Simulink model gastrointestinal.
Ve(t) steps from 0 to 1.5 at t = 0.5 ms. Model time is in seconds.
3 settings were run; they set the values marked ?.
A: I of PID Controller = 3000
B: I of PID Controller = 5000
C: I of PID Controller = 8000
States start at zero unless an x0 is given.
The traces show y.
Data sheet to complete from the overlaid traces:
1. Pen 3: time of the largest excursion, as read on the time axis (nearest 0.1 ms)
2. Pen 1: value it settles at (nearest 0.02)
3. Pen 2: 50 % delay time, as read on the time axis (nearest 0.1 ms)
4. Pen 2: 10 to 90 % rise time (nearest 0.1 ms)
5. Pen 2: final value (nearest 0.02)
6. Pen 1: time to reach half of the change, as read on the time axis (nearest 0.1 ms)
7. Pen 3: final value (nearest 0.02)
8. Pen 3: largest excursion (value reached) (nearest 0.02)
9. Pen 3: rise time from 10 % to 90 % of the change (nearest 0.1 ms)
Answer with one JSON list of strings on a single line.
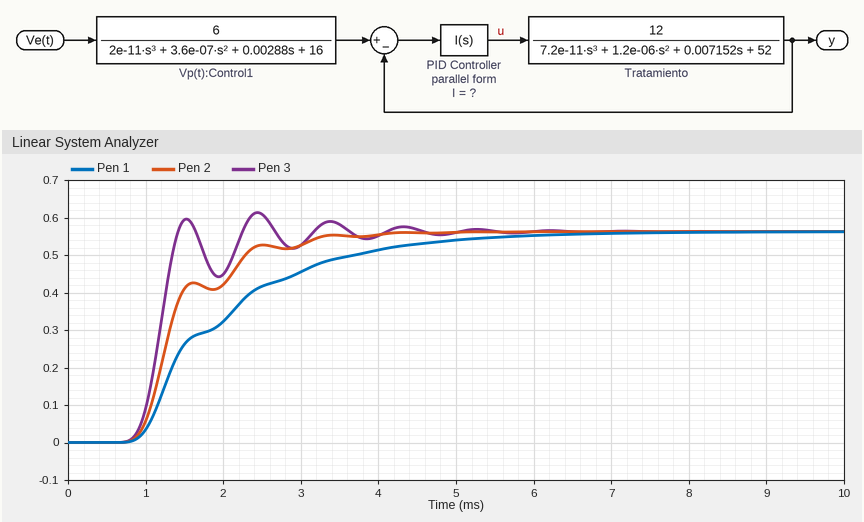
["2.4 ms", "0.56", "1.3 ms", "1.3 ms", "0.56", "1.6 ms", "0.56", "0.62", "0.4 ms"]
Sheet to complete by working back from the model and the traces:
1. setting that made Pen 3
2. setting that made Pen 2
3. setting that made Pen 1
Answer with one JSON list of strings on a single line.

["C", "B", "A"]
